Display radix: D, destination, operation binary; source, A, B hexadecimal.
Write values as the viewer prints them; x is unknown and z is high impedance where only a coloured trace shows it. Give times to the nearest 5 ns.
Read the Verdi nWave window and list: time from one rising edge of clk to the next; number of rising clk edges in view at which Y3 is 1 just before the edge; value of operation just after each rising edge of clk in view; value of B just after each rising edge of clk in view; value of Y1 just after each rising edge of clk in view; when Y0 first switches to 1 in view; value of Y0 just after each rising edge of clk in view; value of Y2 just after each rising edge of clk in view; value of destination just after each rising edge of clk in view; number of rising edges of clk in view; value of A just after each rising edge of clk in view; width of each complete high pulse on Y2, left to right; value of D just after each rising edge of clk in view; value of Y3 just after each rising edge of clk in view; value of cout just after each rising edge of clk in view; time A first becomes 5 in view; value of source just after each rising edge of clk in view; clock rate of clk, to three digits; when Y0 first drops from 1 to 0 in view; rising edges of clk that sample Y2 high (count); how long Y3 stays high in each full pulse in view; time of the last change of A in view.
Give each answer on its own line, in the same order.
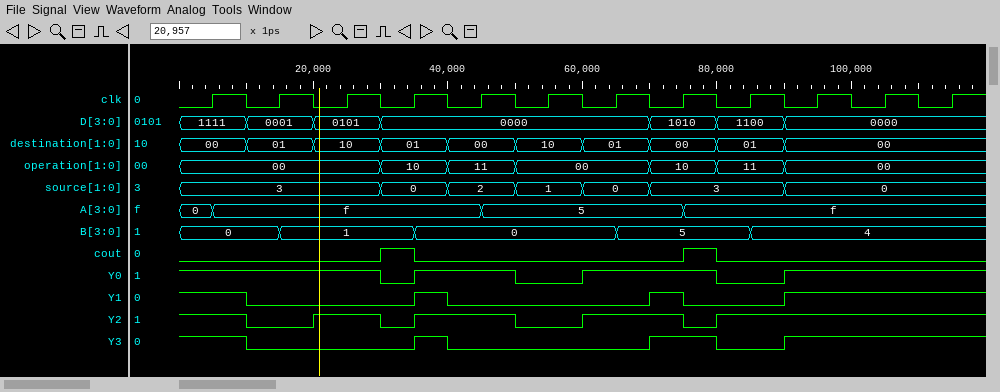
10 ns
5
00, 00, 00, 10, 11, 00, 00, 10, 11, 00, 00, 00
0, 1, 1, 0, 0, 0, 5, 5, 4, 4, 4, 4
1 0 0 1 0 0 0 0 0 1 1 1
35 ns
1 1 1 1 1 0 1 1 0 1 1 1
1 0 1 1 1 0 1 0 1 1 1 1
00, 01, 10, 01, 00, 10, 01, 00, 01, 00, 00, 00
12
f, f, f, f, 5, 5, 5, f, f, f, f, f
10 ns, 15 ns, 15 ns
1111, 0001, 0101, 0000, 0000, 0000, 0000, 1010, 1100, 0000, 0000, 0000
1 0 0 1 0 0 0 1 0 1 1 1
0 0 0 0 0 0 0 1 0 0 0 0
45 ns
3, 3, 3, 0, 2, 1, 0, 3, 3, 0, 0, 0
100 MHz
30 ns
9
5 ns, 10 ns
75 ns
